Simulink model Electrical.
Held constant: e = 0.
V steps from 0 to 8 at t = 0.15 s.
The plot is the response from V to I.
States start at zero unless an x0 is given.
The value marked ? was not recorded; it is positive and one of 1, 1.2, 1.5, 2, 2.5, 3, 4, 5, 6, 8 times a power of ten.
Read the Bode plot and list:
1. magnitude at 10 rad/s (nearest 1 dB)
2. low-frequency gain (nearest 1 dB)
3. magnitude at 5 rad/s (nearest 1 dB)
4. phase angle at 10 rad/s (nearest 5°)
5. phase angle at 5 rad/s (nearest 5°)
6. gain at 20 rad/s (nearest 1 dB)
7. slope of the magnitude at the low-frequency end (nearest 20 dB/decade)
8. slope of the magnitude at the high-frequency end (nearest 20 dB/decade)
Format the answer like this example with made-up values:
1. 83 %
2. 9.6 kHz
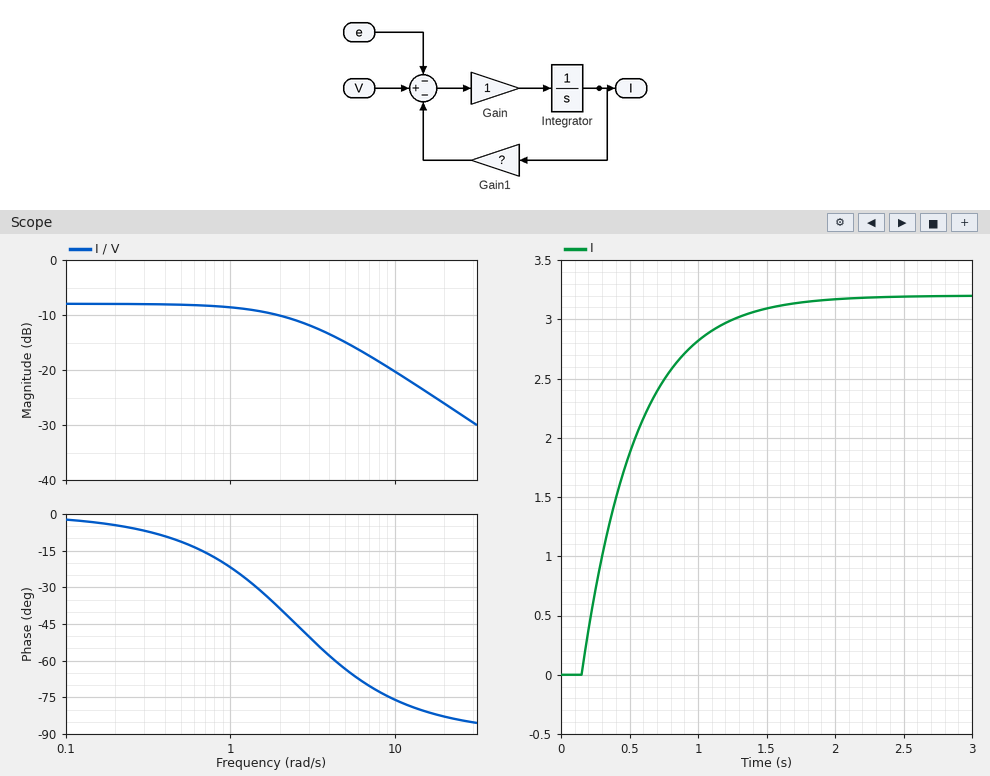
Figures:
1. -20 dB
2. -8 dB
3. -15 dB
4. -75°
5. -65°
6. -26 dB
7. 0 dB/decade
8. -20 dB/decade
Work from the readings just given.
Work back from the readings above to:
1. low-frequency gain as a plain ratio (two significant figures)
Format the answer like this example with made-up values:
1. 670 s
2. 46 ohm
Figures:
1. 0.40
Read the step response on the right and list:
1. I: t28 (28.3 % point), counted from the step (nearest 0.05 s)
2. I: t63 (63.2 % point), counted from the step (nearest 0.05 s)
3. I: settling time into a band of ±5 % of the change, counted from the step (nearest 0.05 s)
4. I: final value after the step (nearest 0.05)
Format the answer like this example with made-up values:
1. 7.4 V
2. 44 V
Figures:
1. 0.15 s
2. 0.40 s
3. 1.20 s
4. 3.20
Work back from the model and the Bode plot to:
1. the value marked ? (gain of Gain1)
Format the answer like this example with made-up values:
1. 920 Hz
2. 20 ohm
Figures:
1. 2.5
